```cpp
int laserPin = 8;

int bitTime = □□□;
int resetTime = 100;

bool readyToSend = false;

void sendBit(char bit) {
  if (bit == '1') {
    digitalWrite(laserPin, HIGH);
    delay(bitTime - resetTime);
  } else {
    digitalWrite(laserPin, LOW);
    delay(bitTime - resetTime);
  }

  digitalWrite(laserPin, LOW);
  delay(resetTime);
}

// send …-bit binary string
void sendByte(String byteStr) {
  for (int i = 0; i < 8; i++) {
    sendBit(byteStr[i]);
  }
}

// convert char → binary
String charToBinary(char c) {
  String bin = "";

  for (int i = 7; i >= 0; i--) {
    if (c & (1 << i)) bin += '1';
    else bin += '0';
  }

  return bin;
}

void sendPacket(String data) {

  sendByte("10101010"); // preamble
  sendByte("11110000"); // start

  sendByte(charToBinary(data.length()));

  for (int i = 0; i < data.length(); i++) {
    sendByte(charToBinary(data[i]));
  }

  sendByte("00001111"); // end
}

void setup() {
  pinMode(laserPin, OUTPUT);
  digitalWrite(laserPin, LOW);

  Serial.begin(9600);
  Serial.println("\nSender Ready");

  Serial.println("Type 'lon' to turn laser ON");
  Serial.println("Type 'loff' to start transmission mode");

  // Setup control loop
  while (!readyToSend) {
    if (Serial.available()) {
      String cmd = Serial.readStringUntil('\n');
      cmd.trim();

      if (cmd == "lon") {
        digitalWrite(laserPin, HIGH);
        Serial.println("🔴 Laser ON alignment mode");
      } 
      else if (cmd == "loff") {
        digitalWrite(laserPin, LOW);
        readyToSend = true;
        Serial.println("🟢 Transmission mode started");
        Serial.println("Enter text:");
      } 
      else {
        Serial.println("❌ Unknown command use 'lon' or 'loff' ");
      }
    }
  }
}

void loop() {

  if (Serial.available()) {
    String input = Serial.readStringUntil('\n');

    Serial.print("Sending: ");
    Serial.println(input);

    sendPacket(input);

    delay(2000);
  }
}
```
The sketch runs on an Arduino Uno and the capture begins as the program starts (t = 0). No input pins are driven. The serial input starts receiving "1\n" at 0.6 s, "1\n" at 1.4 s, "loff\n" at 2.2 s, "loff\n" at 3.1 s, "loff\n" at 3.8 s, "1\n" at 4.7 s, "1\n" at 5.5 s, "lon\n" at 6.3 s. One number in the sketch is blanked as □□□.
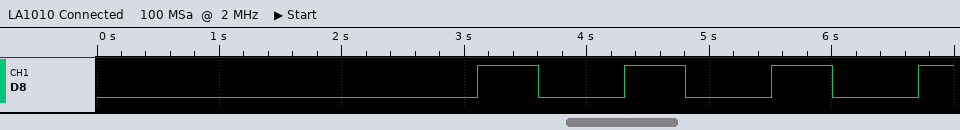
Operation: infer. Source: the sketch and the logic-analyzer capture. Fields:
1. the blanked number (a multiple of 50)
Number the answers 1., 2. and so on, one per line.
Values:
1. 600
